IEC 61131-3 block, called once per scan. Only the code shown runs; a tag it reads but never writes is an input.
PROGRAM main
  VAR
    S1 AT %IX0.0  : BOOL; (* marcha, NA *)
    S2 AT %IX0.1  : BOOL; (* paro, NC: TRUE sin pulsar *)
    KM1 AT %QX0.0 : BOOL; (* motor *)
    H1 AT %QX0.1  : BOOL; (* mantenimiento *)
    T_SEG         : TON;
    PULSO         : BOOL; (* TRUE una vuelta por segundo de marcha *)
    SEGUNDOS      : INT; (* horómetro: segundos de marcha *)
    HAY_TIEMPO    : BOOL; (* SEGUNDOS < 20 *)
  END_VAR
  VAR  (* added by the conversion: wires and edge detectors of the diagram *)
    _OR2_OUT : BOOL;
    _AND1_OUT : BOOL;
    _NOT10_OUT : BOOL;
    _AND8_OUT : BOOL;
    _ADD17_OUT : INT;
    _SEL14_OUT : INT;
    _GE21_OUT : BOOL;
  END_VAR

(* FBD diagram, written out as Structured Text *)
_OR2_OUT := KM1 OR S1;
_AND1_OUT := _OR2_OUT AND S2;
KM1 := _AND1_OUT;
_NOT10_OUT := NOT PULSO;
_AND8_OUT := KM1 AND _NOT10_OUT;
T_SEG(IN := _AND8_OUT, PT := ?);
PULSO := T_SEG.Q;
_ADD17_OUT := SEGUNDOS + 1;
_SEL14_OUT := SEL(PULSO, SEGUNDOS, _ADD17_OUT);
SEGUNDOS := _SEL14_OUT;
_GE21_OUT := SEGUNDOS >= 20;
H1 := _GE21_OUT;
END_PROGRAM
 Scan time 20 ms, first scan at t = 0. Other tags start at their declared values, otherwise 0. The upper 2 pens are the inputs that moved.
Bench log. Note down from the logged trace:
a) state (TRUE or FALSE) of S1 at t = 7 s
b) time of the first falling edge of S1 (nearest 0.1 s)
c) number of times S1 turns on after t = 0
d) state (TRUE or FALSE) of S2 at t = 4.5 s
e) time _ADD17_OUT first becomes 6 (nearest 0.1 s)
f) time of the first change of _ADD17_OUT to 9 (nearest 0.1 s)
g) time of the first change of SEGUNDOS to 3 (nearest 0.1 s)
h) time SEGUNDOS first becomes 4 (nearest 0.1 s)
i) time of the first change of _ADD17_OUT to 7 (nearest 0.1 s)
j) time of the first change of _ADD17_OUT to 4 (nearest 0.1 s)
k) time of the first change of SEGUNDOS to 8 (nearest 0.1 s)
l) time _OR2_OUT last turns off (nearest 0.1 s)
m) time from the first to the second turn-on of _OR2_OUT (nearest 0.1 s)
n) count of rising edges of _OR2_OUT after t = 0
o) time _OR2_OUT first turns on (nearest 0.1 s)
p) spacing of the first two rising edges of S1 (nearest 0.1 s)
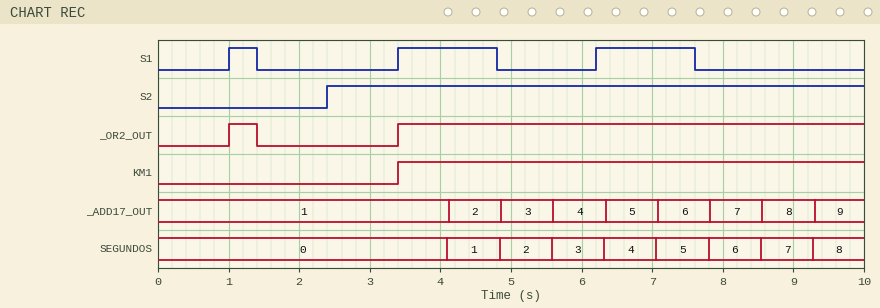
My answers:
TRUE
1.4 s
3
TRUE
7.1 s
9.3 s
5.6 s
6.3 s
7.8 s
5.6 s
9.3 s
1.4 s
2.4 s
2
1.0 s
2.4 s
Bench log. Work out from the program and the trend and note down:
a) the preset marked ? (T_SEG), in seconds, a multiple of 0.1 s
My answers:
0.7 s
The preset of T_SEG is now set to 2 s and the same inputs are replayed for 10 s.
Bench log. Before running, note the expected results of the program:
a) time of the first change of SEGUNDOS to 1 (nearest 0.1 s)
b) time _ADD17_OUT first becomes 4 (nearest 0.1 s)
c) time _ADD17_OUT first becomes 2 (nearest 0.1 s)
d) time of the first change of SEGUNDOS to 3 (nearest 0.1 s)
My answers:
5.4 s
9.5 s
5.4 s
9.5 s
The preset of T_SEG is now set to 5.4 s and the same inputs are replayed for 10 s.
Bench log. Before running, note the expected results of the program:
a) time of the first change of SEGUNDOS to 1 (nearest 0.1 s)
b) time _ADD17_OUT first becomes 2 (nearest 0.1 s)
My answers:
8.8 s
8.8 s
